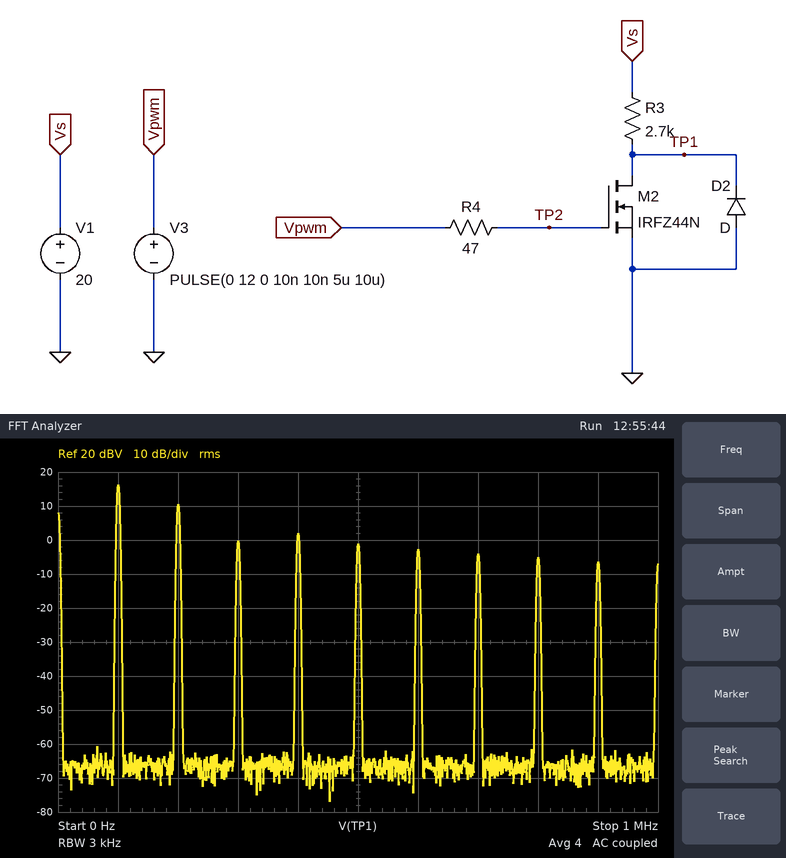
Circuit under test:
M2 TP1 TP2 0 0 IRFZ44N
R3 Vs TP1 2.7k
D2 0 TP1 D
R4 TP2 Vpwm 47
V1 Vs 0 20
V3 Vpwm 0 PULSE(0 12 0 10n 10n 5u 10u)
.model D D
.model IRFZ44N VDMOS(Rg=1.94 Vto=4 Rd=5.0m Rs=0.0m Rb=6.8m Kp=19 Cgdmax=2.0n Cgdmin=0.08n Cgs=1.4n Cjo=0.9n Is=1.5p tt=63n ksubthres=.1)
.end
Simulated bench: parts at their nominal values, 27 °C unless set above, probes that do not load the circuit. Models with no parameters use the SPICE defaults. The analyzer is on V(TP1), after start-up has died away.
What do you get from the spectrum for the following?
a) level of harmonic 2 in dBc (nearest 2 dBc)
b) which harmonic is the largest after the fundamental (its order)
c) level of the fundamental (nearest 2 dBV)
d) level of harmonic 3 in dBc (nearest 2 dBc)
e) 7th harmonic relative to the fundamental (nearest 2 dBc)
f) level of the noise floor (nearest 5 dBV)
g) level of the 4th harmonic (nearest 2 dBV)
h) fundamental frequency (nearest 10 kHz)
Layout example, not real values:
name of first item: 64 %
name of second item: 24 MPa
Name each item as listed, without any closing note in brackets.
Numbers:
level of harmonic 2 in dBc: -6 dBc
which harmonic is the largest after the fundamental: 2
level of the fundamental: 16 dBV
level of harmonic 3 in dBc: -16 dBc
7th harmonic relative to the fundamental: -20 dBc
level of the noise floor: -65 dBV
level of the 4th harmonic: 2 dBV
fundamental frequency: 100 kHz
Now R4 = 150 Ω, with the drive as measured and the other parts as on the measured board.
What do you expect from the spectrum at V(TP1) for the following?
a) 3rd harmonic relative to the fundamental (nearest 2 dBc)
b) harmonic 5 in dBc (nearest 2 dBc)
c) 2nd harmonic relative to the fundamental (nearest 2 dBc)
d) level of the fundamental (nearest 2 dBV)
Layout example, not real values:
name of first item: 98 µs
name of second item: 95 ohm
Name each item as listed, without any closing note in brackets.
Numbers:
3rd harmonic relative to the fundamental: -12 dBc
harmonic 5 in dBc: -16 dBc
2nd harmonic relative to the fundamental: -4 dBc
level of the fundamental: 14 dBV
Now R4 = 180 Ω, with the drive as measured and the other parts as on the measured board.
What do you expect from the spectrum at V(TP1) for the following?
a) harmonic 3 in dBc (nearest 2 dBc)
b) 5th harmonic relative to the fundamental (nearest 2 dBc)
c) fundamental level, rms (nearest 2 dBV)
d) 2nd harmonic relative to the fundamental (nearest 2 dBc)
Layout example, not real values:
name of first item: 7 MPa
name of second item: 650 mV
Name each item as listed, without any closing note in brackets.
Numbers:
harmonic 3 in dBc: -10 dBc
5th harmonic relative to the fundamental: -16 dBc
fundamental level, rms: 14 dBV
2nd harmonic relative to the fundamental: -4 dBc
